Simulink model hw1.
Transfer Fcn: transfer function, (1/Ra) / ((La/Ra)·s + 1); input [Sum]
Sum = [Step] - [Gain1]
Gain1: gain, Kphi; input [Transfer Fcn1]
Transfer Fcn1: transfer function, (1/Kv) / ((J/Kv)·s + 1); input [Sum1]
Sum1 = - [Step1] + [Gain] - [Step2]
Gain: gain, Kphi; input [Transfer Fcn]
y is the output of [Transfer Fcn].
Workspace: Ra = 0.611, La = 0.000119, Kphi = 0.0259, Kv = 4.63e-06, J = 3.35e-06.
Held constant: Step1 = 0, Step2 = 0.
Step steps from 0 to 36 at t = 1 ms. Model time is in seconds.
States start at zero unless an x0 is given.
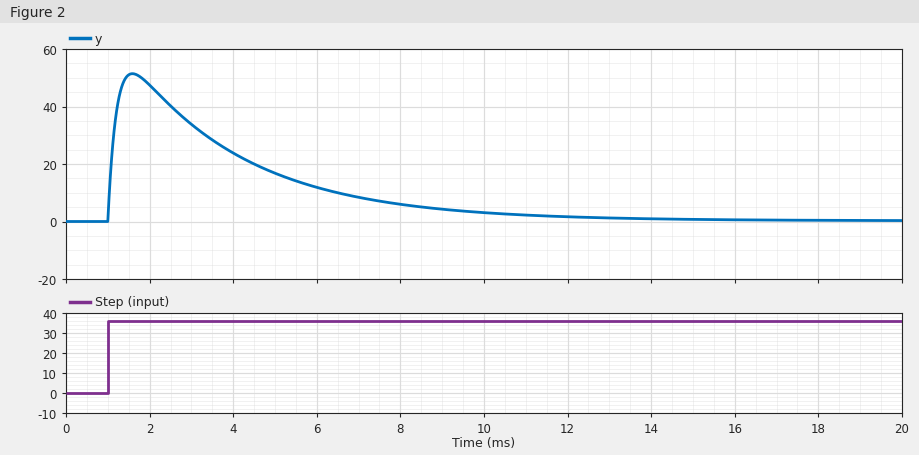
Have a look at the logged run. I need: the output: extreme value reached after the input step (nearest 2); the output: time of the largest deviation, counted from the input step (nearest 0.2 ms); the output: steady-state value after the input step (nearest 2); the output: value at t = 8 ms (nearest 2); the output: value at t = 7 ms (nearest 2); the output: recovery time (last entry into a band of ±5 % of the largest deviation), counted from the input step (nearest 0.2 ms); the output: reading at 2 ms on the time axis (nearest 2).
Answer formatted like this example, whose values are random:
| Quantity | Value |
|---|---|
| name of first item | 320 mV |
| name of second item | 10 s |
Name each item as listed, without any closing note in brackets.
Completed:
| Quantity | Value |
|---|---|
| the output: extreme value reached after the input step | 52 |
| the output: time of the largest deviation, counted from the input step | 0.6 ms |
| the output: steady-state value after the input step | 0 |
| the output: value at t = 8 ms | 6 |
| the output: value at t = 7 ms | 8 |
| the output: recovery time (last entry into a band of ±5 % of the largest deviation), counted from the input step | 9.2 ms |
| the output: reading at 2 ms on the time axis | 48 |
